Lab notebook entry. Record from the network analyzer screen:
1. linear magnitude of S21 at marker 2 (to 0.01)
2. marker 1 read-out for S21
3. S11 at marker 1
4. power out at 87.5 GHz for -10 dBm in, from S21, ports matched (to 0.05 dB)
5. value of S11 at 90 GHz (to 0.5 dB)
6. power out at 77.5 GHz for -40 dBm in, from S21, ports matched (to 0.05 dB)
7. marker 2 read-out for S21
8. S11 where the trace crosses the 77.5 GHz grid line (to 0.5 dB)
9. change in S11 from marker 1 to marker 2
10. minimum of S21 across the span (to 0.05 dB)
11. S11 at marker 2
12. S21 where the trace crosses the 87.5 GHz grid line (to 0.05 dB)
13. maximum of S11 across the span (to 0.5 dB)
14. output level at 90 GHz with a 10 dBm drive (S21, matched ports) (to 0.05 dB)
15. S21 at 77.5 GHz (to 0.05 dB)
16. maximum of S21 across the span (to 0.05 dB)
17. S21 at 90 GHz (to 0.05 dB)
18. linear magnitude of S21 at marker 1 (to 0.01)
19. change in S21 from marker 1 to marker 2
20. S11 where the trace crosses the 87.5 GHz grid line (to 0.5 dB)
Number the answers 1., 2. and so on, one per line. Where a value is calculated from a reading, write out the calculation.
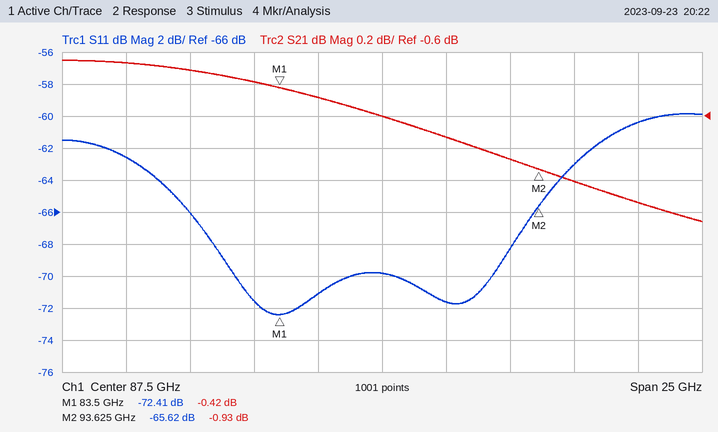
1. 10^(-0.93/20) ≈ 0.90
2. -0.42 dB
3. -72.41 dB
4. -10 dBm + (-0.60 dB) = -10.60 dBm
5. -71.5 dB
6. -40 dBm + (-0.25 dB) = -40.25 dBm
7. -0.93 dB
8. -62.5 dB
9. -65.62 − (-72.41) = 6.79 dB
10. -1.25 dB
11. -65.62 dB
12. -0.60 dB
13. -60.0 dB
14. 10 dBm + (-0.75 dB) = 9.25 dBm
15. -0.25 dB
16. -0.25 dB
17. -0.75 dB
18. 10^(-0.42/20) ≈ 0.95
19. -0.93 − (-0.42) = -0.51 dB
20. -70.0 dB
